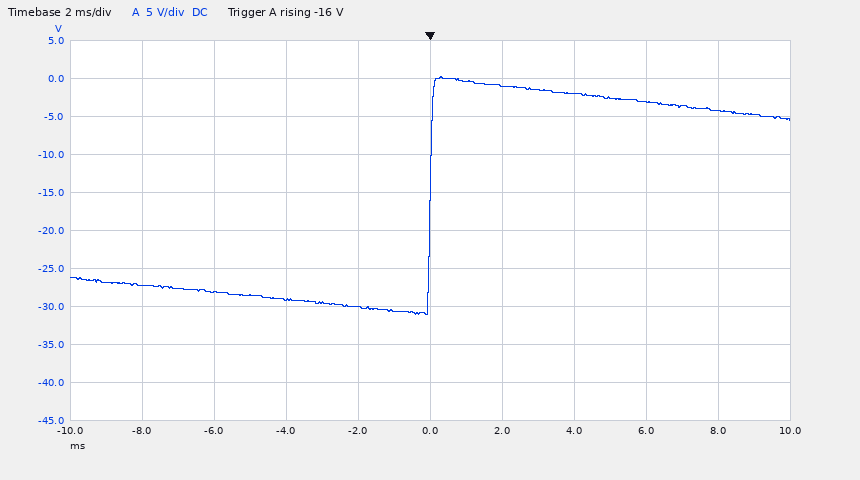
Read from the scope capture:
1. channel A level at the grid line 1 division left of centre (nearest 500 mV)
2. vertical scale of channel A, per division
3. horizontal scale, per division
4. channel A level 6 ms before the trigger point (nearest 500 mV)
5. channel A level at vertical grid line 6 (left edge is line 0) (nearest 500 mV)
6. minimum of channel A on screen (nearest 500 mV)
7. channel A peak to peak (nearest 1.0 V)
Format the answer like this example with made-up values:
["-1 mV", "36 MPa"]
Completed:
["-30.0 V", "5 V", "2 ms", "-28.0 V", "-1.0 V", "-31.0 V", "31.0 V"]
